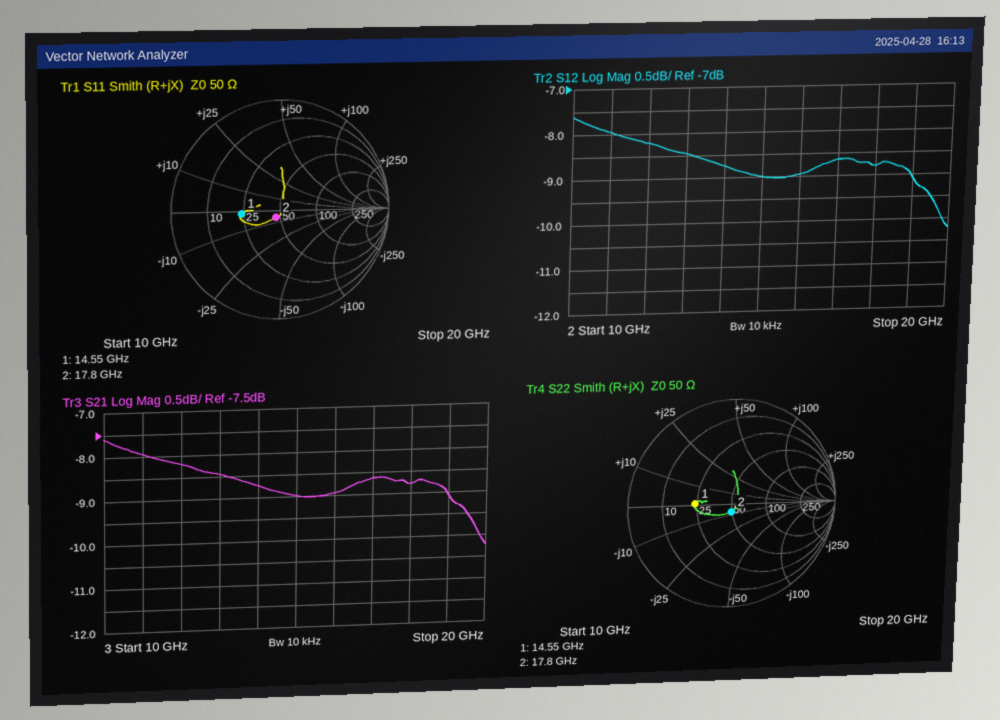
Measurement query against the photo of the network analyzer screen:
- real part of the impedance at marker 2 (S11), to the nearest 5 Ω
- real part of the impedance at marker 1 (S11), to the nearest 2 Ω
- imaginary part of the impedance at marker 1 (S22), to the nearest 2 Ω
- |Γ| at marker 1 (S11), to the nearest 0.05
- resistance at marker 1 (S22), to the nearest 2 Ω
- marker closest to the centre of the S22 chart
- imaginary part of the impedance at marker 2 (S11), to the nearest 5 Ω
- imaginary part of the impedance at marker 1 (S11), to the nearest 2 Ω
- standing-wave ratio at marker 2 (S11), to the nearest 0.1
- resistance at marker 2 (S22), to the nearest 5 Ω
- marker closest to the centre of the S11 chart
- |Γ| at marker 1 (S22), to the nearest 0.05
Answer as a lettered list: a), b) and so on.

a) 45 Ω
b) 24 Ω
c) 0 Ω
d) 0.35
e) 24 Ω
f) marker 2
g) -5 Ω
h) -2 Ω
i) 1.2
j) 50 Ω
k) marker 2
l) 0.35
